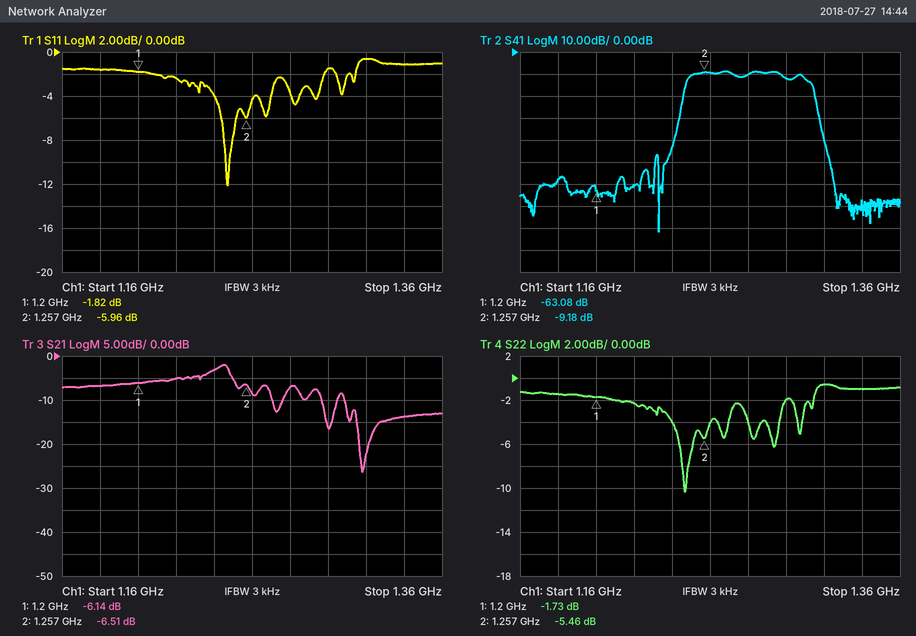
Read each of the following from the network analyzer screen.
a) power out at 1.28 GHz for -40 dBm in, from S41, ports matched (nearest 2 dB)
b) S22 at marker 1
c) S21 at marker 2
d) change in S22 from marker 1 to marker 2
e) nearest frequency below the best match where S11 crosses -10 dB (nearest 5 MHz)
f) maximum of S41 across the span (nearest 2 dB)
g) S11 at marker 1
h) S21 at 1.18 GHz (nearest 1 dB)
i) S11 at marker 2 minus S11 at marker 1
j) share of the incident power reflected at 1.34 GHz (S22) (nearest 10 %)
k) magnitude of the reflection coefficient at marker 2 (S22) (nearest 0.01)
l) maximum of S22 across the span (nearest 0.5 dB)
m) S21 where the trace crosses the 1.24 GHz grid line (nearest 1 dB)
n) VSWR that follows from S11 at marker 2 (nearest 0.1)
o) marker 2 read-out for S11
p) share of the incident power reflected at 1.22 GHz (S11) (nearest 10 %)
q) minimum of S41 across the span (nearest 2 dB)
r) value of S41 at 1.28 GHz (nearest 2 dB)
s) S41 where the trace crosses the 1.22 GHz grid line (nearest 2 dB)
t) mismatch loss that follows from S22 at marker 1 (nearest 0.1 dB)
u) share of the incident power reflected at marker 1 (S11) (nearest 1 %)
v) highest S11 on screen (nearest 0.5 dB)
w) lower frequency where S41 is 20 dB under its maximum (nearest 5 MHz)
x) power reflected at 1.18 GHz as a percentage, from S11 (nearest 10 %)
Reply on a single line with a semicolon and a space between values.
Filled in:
-50 dBm; -1.73 dB; -6.51 dB; -3.73 dB; 1.245 GHz; -8 dB; -1.82 dB; -7 dB; -4.14 dB; 80 %; 0.53; -0.5 dB; -3 dB; 3.0; -5.96 dB; 60 %; -82 dB; -10 dB; -60 dB; 4.8 dB; 66 %; -0.5 dB; 1.245 GHz; 70 %
